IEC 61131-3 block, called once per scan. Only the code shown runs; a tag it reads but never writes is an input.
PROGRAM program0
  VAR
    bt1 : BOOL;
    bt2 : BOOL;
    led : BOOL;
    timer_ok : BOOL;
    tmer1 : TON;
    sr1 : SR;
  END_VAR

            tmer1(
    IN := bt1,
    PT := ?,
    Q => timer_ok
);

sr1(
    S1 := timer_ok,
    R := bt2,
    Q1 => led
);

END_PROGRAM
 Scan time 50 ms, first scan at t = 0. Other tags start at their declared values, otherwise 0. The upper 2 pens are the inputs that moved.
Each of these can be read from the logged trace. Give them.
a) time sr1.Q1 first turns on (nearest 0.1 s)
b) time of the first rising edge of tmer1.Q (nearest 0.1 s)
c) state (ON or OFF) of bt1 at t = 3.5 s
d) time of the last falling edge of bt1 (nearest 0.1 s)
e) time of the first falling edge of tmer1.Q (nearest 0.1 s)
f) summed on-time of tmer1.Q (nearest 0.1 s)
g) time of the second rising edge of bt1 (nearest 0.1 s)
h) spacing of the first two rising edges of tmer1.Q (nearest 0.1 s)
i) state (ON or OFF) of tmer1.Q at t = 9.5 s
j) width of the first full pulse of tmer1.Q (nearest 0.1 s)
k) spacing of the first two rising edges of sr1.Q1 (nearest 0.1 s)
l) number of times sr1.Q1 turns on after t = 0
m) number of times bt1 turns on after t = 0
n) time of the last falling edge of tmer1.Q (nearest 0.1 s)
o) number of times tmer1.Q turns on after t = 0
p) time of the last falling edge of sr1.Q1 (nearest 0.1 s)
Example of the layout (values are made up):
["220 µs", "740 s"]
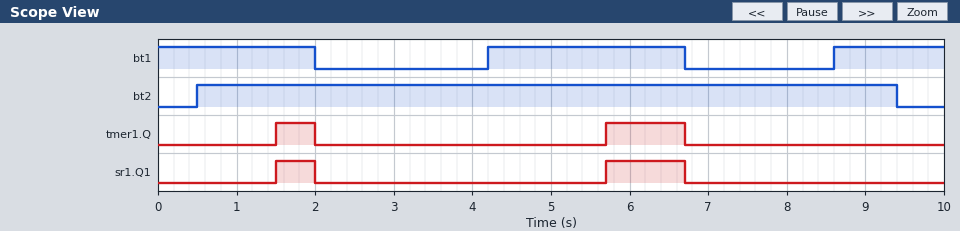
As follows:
["1.5 s", "1.5 s", "OFF", "6.7 s", "2.0 s", "1.5 s", "8.6 s", "4.2 s", "OFF", "0.5 s", "4.2 s", "2", "2", "6.7 s", "2", "6.7 s"]
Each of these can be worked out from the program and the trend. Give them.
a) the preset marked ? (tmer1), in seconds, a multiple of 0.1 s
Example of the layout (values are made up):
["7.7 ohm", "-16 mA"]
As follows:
["1.5 s"]
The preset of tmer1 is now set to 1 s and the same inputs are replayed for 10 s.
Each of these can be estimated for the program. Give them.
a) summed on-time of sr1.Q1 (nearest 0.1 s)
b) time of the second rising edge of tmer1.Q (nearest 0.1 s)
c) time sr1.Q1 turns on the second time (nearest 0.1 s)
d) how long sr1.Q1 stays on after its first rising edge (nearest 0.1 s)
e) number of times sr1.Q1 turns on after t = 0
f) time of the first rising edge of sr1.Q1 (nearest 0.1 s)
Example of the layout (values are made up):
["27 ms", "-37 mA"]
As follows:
["2.9 s", "5.2 s", "5.2 s", "1.0 s", "3", "1.0 s"]
